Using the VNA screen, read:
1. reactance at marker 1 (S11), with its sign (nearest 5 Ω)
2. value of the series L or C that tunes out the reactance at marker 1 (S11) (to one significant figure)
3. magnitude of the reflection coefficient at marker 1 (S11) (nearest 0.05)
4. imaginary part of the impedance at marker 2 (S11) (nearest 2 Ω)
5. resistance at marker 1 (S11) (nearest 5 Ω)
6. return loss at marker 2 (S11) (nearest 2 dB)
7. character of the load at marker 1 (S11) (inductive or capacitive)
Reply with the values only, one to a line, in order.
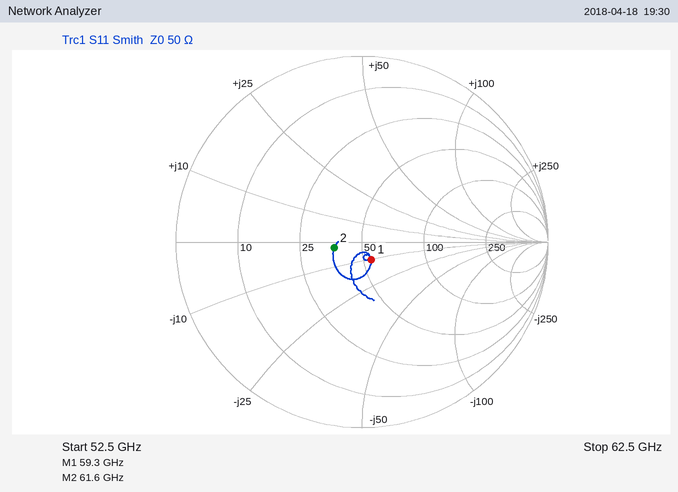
-10 Ω
30 pH
0.10
-2 Ω
55 Ω
16 dB
capacitive
